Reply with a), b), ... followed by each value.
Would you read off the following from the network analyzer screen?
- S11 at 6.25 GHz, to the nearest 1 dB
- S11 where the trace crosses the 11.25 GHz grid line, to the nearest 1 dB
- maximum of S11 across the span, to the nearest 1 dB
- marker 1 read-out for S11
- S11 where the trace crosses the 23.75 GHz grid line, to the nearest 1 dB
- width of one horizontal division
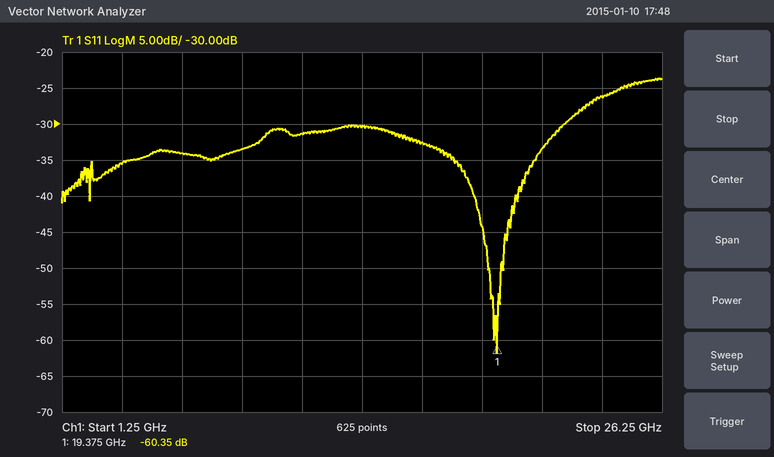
a) -34 dB
b) -31 dB
c) -24 dB
d) -60.35 dB
e) -26 dB
f) 2.5 GHz
